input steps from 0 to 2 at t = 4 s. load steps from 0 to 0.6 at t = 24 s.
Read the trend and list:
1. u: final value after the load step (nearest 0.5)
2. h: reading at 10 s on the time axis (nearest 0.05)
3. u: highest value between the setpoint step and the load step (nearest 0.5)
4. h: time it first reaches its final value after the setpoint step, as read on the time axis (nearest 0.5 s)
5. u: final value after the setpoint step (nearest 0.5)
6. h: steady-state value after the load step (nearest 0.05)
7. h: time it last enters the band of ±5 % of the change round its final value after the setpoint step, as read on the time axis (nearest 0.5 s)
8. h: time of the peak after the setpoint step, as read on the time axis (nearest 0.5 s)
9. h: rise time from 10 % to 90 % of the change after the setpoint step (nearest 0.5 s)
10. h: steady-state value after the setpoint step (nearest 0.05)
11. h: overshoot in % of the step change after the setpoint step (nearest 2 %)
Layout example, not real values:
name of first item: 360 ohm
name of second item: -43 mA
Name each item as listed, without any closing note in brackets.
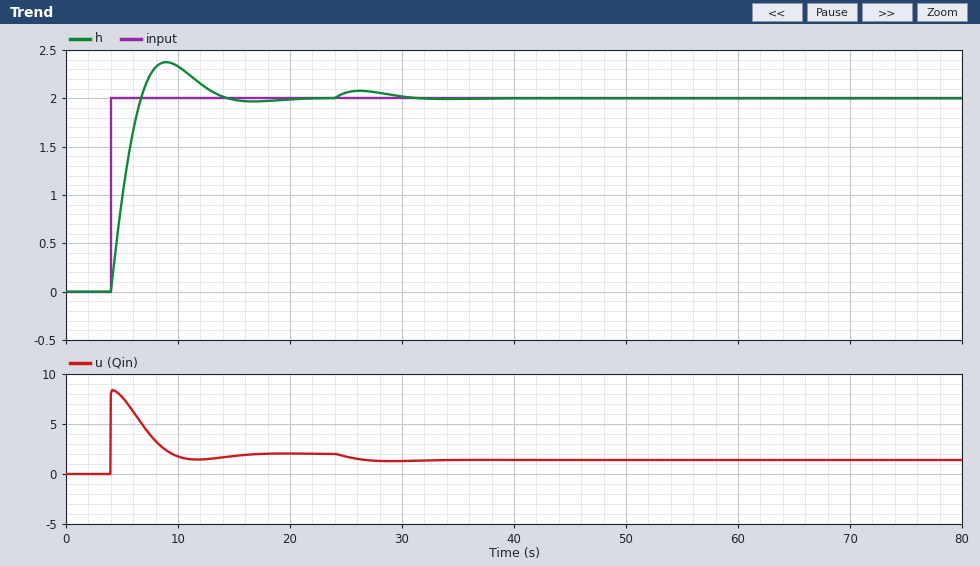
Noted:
u: final value after the load step: 1.5
h: reading at 10 s on the time axis: 2.35
u: highest value between the setpoint step and the load step: 8.5
h: time it first reaches its final value after the setpoint step, as read on the time axis: 6.5 s
u: final value after the setpoint step: 2.0
h: steady-state value after the load step: 2.00
h: time it last enters the band of ±5 % of the change round its final value after the setpoint step, as read on the time axis: 12.5 s
h: time of the peak after the setpoint step, as read on the time axis: 9.0 s
h: rise time from 10 % to 90 % of the change after the setpoint step: 2.0 s
h: steady-state value after the setpoint step: 2.00
h: overshoot in % of the step change after the setpoint step: 18 %
